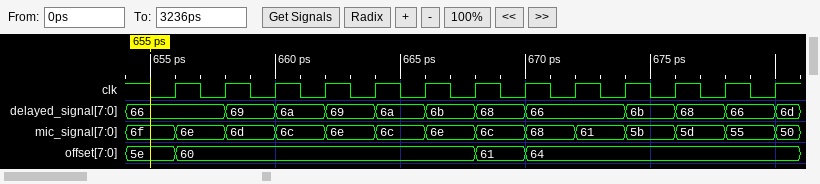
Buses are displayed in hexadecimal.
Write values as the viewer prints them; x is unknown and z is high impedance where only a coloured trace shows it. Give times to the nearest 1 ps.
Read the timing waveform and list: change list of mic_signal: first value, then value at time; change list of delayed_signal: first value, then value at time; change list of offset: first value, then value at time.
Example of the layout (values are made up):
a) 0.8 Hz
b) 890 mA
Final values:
a) 6f, 6e at 656 ps, 6d at 658 ps, 6c at 660 ps, 6e at 662 ps, 6c at 664 ps, 6e at 666 ps, 6c at 668 ps, 68 at 670 ps, 61 at 672 ps, 5b at 674 ps, 5d at 676 ps, 55 at 678 ps, 50 at 680 ps
b) 66, 69 at 658 ps, 6a at 660 ps, 69 at 662 ps, 6a at 664 ps, 6b at 666 ps, 68 at 668 ps, 66 at 670 ps, 6b at 674 ps, 68 at 676 ps, 66 at 678 ps, 6d at 680 ps
c) 5e, 60 at 656 ps, 61 at 668 ps, 64 at 670 ps
